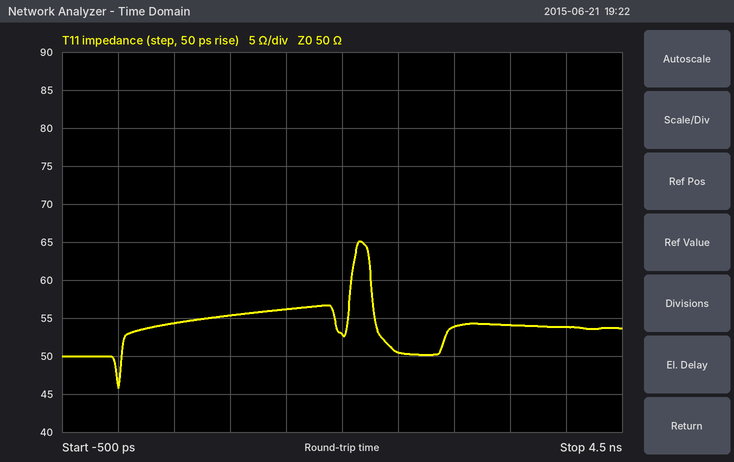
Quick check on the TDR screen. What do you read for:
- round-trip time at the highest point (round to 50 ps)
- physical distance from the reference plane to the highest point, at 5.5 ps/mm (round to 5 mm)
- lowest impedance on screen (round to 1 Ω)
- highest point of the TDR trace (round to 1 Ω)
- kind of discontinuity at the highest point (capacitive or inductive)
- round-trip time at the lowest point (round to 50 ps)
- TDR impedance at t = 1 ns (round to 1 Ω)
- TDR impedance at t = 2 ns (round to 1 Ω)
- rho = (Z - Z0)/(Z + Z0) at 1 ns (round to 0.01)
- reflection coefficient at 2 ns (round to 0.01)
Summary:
2.15 ns
195 mm
46 Ω
65 Ω
inductive
0 ps
55 Ω
53 Ω
+0.05
+0.03
